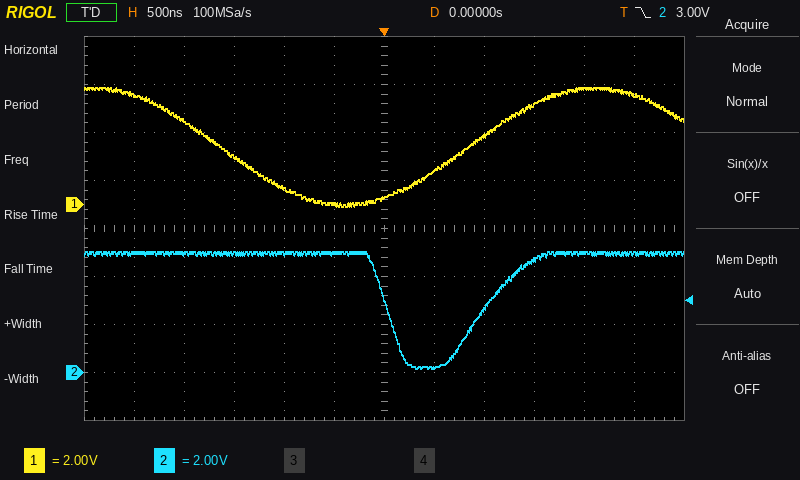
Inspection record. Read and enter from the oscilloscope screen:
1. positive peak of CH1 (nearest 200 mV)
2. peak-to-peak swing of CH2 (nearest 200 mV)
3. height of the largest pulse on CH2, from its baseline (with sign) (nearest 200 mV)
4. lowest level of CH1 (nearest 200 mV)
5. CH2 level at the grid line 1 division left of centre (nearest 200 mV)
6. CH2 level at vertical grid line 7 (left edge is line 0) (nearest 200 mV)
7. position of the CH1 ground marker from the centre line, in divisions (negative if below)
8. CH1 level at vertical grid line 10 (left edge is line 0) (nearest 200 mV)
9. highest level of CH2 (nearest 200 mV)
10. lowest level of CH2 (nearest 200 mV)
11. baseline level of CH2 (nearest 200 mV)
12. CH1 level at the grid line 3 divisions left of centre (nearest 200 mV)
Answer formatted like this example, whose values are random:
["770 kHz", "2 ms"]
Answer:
["4.8 V", "4.8 V", "-4.8 V", "0.0 V", "5.0 V", "200 mV", "+0.5 div", "4.8 V", "5.0 V", "200 mV", "5.0 V", "2.0 V"]
